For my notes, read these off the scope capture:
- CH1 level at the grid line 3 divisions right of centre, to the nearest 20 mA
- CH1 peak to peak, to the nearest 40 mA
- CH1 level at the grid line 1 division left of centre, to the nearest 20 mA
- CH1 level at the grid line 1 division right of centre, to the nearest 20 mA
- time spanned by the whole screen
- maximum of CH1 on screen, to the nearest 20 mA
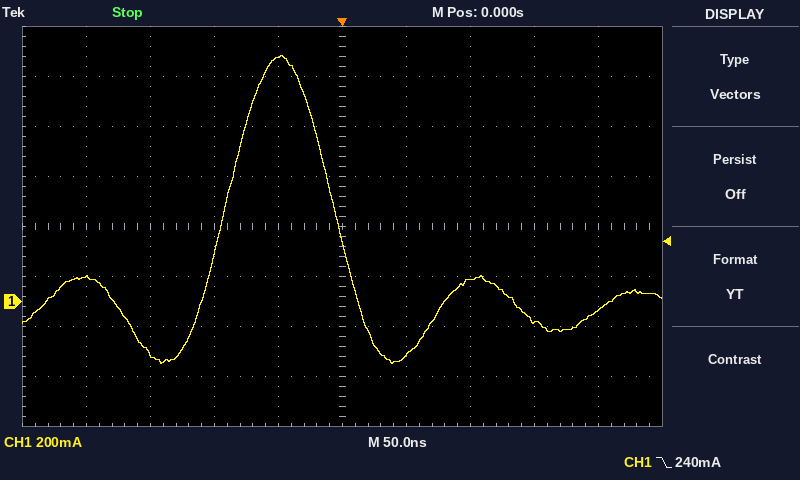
-80 mA
1.24 A
980 mA
-220 mA
500 ns
980 mA
